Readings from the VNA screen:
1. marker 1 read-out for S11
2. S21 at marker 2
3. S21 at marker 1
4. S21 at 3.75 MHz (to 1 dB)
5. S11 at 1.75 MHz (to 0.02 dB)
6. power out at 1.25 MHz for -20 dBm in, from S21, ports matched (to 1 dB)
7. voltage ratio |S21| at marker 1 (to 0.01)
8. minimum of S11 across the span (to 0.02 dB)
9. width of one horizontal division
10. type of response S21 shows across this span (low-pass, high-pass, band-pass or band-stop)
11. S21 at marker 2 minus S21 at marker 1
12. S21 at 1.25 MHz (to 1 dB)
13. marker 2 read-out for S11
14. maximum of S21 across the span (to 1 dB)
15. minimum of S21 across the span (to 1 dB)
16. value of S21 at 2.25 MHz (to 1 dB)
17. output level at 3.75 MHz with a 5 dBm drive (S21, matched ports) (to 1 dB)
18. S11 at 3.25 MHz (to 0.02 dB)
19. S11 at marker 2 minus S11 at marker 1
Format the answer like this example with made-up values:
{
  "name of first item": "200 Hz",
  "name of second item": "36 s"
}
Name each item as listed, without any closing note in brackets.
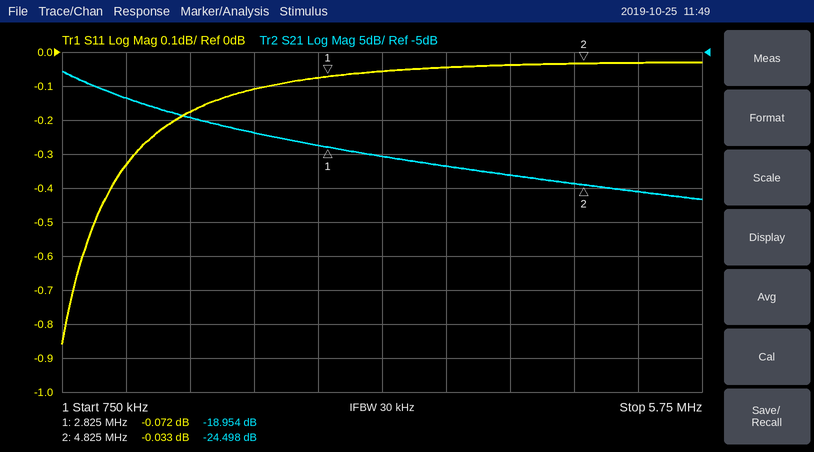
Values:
{
  "marker 1 read-out for S11": "-0.072 dB",
  "S21 at marker 2": "-24.498 dB",
  "S21 at marker 1": "-18.954 dB",
  "S21 at 3.75 MHz": "-22 dB",
  "S11 at 1.75 MHz": "-0.18 dB",
  "power out at 1.25 MHz for -20 dBm in, from S21, ports matched": "-32 dBm",
  "voltage ratio |S21| at marker 1": "0.11",
  "minimum of S11 across the span": "-0.86 dB",
  "width of one horizontal division": "500 kHz",
  "type of response S21 shows across this span": "low-pass",
  "S21 at marker 2 minus S21 at marker 1": "-5.544 dB",
  "S21 at 1.25 MHz": "-12 dB",
  "marker 2 read-out for S11": "-0.033 dB",
  "maximum of S21 across the span": "-8 dB",
  "minimum of S21 across the span": "-27 dB",
  "value of S21 at 2.25 MHz": "-17 dB",
  "output level at 3.75 MHz with a 5 dBm drive (S21, matched ports)": "-17 dBm",
  "S11 at 3.25 MHz": "-0.06 dB",
  "S11 at marker 2 minus S11 at marker 1": "0.039 dB"
}
